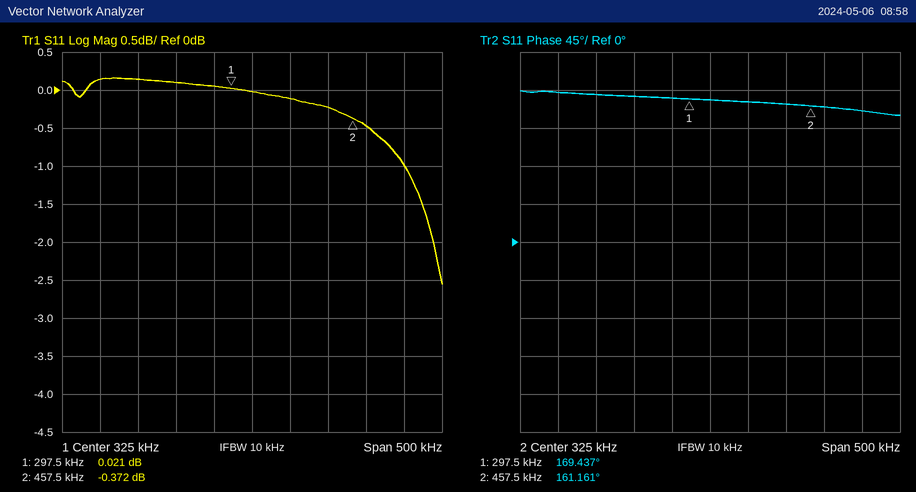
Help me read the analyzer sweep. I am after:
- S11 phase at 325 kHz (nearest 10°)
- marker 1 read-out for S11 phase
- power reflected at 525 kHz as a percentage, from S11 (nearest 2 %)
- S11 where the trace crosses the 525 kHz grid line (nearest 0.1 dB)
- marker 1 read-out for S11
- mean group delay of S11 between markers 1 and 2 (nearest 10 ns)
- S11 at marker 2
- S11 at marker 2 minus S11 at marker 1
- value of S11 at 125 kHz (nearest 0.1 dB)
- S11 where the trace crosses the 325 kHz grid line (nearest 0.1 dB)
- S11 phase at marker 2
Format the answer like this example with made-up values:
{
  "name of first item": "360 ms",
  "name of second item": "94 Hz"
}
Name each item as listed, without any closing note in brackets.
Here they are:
{
  "S11 phase at 325 kHz": "170°",
  "marker 1 read-out for S11 phase": "169.437°",
  "power reflected at 525 kHz as a percentage, from S11": "80 %",
  "S11 where the trace crosses the 525 kHz grid line": "-1.0 dB",
  "marker 1 read-out for S11": "0.021 dB",
  "mean group delay of S11 between markers 1 and 2": "140 ns",
  "S11 at marker 2": "-0.372 dB",
  "S11 at marker 2 minus S11 at marker 1": "-0.393 dB",
  "value of S11 at 125 kHz": "0.1 dB",
  "S11 where the trace crosses the 325 kHz grid line": "0.0 dB",
  "S11 phase at marker 2": "161.161°"
}
